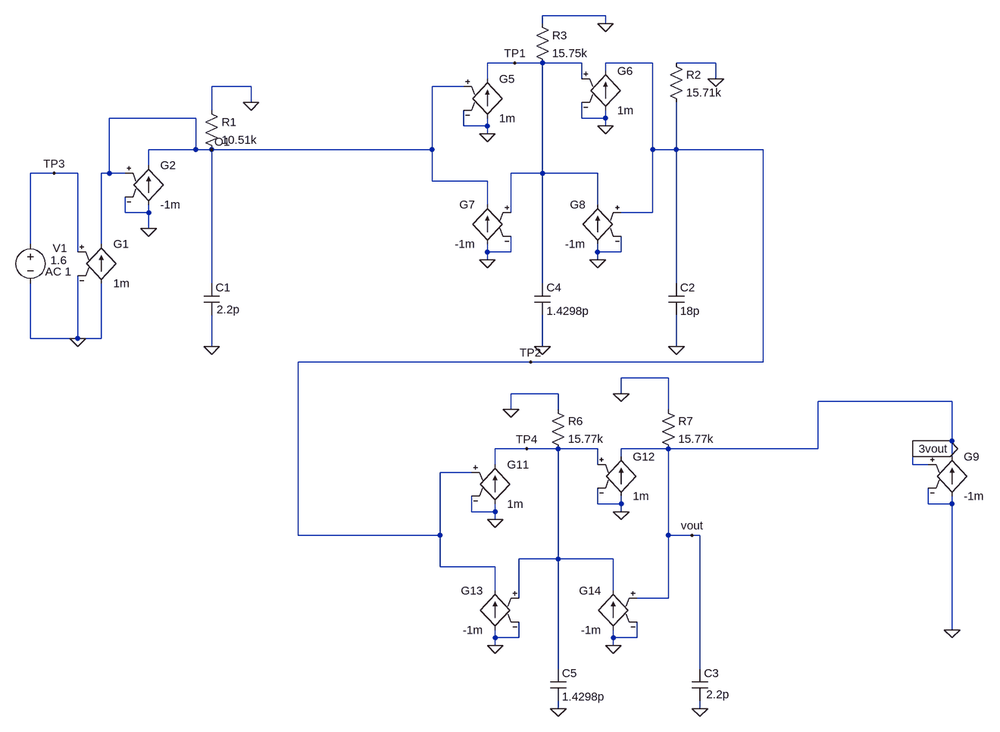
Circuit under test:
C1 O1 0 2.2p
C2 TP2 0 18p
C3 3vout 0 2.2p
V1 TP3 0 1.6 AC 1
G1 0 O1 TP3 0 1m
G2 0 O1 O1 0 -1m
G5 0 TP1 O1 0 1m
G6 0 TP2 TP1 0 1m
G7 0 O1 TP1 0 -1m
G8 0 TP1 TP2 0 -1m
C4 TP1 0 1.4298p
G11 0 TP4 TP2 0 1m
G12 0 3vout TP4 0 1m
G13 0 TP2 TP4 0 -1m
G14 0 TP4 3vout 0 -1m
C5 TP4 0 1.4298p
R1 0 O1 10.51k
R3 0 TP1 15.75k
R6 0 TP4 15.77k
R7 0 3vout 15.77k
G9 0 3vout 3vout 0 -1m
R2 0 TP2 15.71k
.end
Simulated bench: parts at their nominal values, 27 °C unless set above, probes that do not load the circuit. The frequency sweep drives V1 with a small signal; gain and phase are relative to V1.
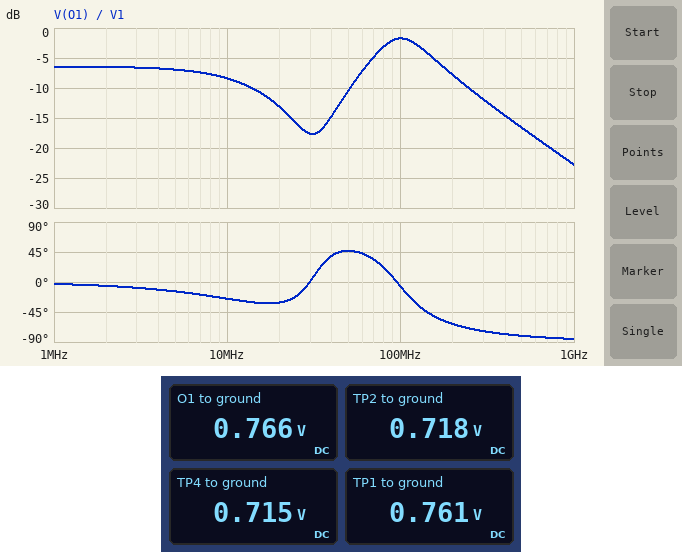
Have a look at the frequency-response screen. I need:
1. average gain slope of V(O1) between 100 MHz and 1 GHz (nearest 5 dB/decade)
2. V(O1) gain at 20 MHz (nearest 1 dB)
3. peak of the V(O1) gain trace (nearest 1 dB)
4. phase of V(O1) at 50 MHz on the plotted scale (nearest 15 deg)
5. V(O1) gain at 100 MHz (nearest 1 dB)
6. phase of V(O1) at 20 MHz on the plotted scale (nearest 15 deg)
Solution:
-20 dB/decade
-13 dB
-2 dB
45 deg
-2 dB
-30 deg
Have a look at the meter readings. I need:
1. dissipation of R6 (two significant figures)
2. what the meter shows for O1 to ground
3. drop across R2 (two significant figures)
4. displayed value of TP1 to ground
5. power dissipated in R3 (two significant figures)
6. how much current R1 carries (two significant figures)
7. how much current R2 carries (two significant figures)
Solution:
32 µW
0.766 V
720 mV
0.761 V
37 µW
73 µA
46 µA
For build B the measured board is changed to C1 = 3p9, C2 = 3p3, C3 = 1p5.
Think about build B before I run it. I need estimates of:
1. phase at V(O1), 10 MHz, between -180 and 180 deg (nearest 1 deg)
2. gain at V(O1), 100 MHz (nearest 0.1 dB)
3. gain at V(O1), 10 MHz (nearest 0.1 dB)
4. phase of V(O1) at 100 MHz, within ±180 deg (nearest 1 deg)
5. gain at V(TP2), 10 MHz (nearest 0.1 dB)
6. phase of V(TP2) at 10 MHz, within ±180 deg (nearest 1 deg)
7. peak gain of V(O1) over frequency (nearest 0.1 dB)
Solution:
-9 deg
-8.1 dB
-6.6 dB
-32 deg
-7.1 dB
-15 deg
-6.4 dB
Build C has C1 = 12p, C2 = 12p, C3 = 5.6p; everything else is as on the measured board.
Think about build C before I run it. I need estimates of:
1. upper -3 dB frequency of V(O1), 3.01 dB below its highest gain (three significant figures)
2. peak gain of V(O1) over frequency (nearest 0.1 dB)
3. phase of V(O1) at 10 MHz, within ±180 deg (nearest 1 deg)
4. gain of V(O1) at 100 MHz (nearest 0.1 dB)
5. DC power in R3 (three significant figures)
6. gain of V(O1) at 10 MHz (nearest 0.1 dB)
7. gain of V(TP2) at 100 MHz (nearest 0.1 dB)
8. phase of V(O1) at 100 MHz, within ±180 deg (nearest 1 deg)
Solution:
11.0 MHz
-6.4 dB
-33 deg
-16.0 dB
36.8 µW
-9.0 dB
-29.0 dB
-79 deg
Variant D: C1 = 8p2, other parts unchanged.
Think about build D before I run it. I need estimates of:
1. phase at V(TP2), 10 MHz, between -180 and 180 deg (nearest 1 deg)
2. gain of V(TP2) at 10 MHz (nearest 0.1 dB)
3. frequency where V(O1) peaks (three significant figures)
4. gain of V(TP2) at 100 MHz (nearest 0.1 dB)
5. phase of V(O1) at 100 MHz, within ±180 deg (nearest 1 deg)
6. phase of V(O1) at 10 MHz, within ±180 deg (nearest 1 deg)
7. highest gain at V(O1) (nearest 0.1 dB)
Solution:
-42 deg
-8.8 dB
58.9 MHz
-30.5 dB
-73 deg
-32 deg
-5.2 dB
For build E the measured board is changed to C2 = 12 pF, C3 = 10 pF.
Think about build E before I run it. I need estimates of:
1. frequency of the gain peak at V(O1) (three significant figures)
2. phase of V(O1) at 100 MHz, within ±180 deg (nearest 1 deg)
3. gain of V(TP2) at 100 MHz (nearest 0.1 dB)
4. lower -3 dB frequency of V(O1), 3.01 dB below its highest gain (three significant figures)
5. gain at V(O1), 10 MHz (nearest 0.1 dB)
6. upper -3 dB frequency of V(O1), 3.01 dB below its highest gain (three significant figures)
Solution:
103 MHz
-2 deg
-15.0 dB
79.8 MHz
-8.8 dB
151 MHz
